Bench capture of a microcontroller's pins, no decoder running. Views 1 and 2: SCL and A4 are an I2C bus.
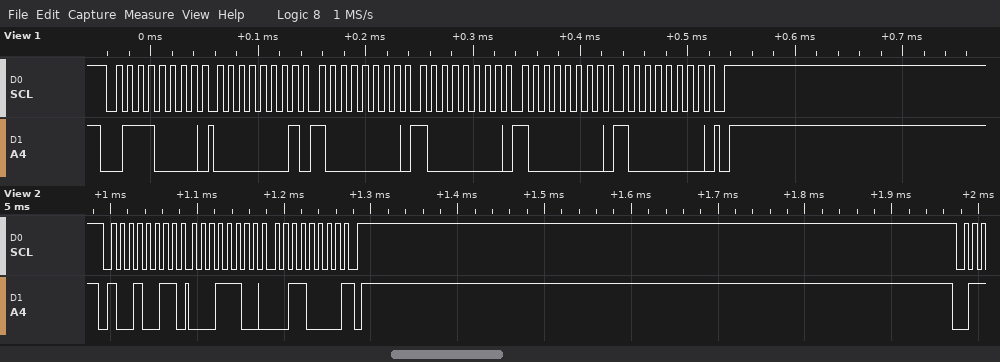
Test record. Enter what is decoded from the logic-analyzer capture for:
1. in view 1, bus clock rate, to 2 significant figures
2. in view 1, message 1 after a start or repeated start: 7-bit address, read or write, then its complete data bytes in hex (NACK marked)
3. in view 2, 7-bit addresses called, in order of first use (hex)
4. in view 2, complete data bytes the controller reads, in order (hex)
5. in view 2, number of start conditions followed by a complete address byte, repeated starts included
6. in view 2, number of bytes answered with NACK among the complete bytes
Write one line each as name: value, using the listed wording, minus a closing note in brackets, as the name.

in view 1, bus clock rate, to 2 significant figures: 100 kHz
in view 1, message 1 after a start or repeated start: 7-bit address, read or write, then its complete data bytes in hex: 0x38 write: 01 80 80 80 80
in view 2, 7-bit addresses called, in order of first use: 0x49
in view 2, complete data bytes the controller reads, in order: 1C 30
in view 2, number of start conditions followed by a complete address byte, repeated starts included: 1
in view 2, number of bytes answered with NACK among the complete bytes: 1
